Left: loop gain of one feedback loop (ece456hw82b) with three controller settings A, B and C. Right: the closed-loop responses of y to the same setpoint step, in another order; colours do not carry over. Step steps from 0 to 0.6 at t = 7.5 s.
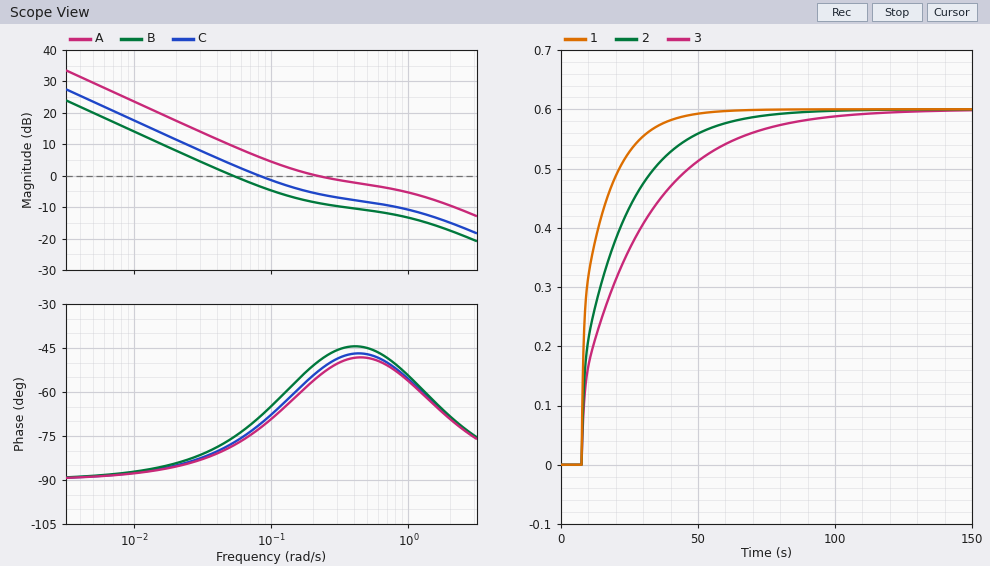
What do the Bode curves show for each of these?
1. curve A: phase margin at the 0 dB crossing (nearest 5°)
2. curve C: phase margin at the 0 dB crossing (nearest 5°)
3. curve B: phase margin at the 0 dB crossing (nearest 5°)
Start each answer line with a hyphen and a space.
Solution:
- 125°
- 110°
- 105°
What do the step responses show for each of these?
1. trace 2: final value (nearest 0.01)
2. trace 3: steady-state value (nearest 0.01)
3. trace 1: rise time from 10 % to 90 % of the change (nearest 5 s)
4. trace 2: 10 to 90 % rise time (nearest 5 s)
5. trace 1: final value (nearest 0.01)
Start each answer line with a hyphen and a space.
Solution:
- 0.60
- 0.60
- 20 s
- 35 s
- 0.60
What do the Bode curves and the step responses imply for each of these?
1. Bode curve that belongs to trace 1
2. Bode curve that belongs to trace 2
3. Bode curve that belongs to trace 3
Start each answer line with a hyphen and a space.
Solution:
- A
- C
- B
